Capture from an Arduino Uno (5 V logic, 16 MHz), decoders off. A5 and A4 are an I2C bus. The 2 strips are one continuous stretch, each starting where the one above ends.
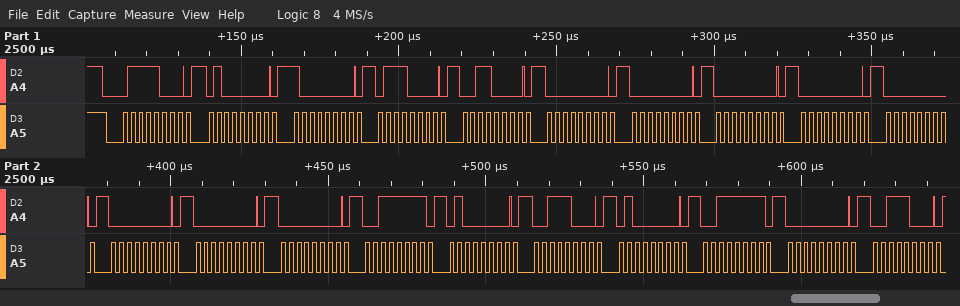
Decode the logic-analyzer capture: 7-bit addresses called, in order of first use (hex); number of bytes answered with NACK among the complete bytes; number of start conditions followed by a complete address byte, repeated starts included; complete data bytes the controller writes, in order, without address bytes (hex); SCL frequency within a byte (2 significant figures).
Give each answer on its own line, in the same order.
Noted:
0x3C
0
1
40 80 70 30 00 00 00 00 00 00 00 00 3F 40 38 40 3F 00 38
400 kHz
